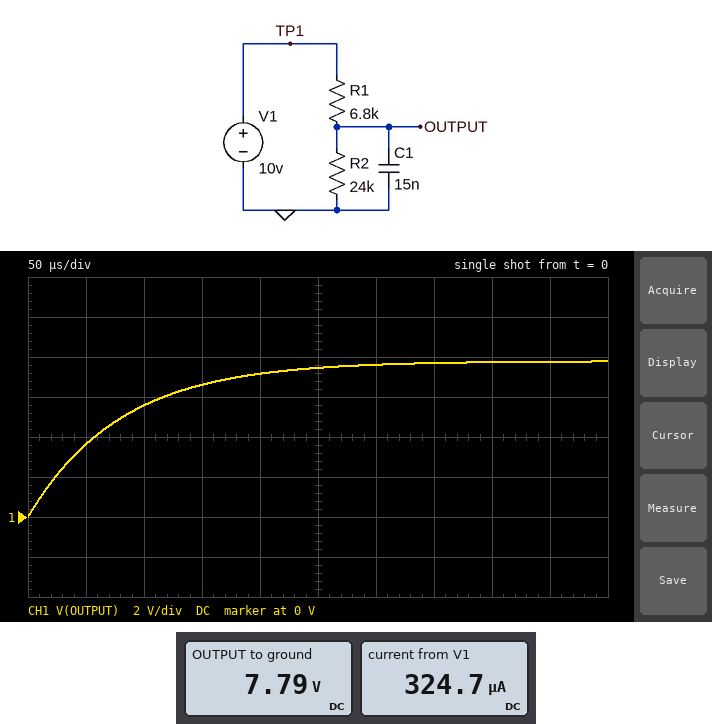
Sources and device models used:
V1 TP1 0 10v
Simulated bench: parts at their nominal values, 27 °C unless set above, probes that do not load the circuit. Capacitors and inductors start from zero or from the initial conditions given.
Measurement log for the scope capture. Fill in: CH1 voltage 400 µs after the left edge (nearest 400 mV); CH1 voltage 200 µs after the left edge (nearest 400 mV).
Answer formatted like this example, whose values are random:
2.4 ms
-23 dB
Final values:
7.6 V
7.2 V
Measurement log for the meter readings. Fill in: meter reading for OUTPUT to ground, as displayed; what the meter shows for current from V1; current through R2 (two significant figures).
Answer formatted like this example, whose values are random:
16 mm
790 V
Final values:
7.79 V
324.7 µA
320 µA
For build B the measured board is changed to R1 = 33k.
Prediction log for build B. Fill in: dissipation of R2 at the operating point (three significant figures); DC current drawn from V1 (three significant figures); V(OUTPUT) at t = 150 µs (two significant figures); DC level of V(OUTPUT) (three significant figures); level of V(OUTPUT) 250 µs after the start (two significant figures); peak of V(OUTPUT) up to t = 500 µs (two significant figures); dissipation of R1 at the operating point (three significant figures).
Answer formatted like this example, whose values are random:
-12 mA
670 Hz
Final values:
739 µW
175 µA
2.2 V
4.21 V
2.9 V
3.8 V
1.02 mW
